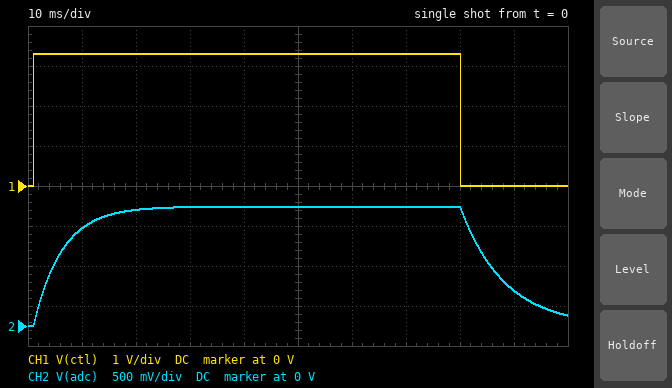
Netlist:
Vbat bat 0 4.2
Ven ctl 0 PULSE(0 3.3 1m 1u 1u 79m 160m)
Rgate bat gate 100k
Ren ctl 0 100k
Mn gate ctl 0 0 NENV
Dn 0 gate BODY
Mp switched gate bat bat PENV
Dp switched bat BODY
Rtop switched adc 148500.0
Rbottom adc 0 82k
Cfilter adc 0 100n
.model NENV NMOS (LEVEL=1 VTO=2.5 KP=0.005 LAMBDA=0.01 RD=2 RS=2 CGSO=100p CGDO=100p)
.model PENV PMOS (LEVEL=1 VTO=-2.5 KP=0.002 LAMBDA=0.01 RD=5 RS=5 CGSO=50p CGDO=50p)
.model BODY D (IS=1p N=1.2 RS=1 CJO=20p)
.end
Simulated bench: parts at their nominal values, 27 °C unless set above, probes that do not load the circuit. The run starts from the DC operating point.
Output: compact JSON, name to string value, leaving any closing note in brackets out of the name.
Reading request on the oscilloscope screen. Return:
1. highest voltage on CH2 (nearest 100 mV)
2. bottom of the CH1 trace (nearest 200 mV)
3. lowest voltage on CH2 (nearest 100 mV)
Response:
{"highest voltage on CH2": "1.5 V", "bottom of the CH1 trace": "0 V", "lowest voltage on CH2": "0 V"}
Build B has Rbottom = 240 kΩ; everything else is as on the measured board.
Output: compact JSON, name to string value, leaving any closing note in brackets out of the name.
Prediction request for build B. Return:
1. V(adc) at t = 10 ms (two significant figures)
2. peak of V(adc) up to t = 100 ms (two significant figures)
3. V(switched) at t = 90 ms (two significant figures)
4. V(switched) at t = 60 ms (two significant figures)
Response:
{"V(adc) at t = 10 ms": "1.6 V", "peak of V(adc) up to t = 100 ms": "2.6 V", "V(switched) at t = 90 ms": "1.7 V", "V(switched) at t = 60 ms": "4.2 V"}
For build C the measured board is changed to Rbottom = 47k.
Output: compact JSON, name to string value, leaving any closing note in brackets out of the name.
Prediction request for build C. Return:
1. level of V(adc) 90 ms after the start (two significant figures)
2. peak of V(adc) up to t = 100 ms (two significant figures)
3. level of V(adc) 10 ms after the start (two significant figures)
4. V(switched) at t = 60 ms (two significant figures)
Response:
{"level of V(adc) 90 ms after the start": "120 mV", "peak of V(adc) up to t = 100 ms": "1.0 V", "level of V(adc) 10 ms after the start": "930 mV", "V(switched) at t = 60 ms": "4.2 V"}
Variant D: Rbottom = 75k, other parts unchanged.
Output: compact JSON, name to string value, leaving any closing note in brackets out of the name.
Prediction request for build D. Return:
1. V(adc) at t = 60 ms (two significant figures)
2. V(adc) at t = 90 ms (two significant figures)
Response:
{"V(adc) at t = 60 ms": "1.4 V", "V(adc) at t = 90 ms": "370 mV"}
